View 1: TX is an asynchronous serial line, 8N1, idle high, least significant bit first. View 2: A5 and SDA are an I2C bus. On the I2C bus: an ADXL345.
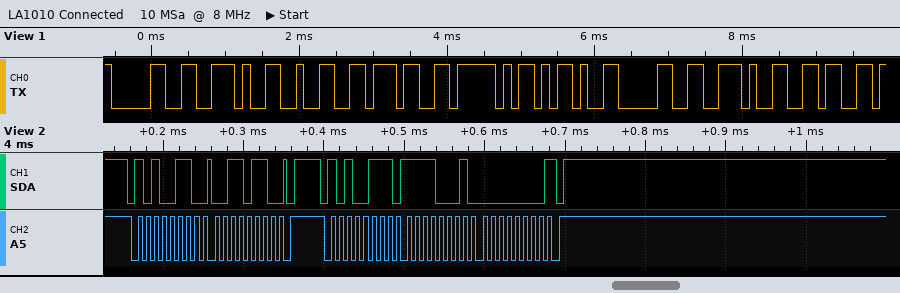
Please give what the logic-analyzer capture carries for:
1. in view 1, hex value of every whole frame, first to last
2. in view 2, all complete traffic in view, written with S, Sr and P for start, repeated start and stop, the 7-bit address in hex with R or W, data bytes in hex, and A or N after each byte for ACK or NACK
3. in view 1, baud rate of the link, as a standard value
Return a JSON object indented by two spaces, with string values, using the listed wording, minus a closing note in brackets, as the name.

{
  "in view 1, hex value of every whole frame, first to last": "30 2E 32 37 5F 2D 30 2E 36",
  "in view 2, all complete traffic in view, written with S, Sr and P for start, repeated start and stop, the 7-bit address in hex with R or W, data bytes in hex, and A or N after each byte for ACK or NACK": "S 53W A 36 A P S 53R A F1 A 00 N P",
  "in view 1, baud rate of the link, as a standard value": "9600 baud"
}
